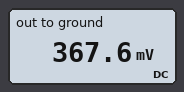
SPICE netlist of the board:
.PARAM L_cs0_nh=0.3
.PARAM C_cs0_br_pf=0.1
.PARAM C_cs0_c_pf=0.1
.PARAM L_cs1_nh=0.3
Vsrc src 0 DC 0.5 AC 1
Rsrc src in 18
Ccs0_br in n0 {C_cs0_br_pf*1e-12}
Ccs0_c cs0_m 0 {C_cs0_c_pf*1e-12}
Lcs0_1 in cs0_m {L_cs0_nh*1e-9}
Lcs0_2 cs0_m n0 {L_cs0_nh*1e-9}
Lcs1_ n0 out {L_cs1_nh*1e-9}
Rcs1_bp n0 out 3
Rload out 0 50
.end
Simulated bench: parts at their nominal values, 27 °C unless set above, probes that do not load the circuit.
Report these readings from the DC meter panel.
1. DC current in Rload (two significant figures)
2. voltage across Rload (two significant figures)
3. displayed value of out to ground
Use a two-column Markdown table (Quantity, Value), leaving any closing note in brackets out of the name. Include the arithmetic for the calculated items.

| Quantity | Value |
|---|---|
| DC current in Rload | (367.6 mV) / 50 Ω = 7.4 mA |
| voltage across Rload | 367.6 mV = 370 mV |
| displayed value of out to ground | 367.6 mV |
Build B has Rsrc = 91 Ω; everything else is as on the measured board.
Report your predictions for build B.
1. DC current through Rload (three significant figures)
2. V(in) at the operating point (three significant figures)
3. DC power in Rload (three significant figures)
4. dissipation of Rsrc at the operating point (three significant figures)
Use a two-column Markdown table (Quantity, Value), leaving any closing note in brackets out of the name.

| Quantity | Value |
|---|---|
| DC current through Rload | 3.55 mA |
| V(in) at the operating point | 177 mV |
| DC power in Rload | 629 µW |
| dissipation of Rsrc at the operating point | 1.14 mW |
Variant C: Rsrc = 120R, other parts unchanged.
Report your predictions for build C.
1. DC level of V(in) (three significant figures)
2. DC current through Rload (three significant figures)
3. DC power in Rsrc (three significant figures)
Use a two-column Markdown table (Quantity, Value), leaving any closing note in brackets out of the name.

| Quantity | Value |
|---|---|
| DC level of V(in) | 147 mV |
| DC current through Rload | 2.94 mA |
| DC power in Rsrc | 1.04 mW |
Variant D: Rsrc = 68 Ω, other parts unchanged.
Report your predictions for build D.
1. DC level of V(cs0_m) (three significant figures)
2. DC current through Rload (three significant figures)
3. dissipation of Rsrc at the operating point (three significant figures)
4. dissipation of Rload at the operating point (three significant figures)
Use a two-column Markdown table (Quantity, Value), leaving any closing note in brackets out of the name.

| Quantity | Value |
|---|---|
| DC level of V(cs0_m) | 212 mV |
| DC current through Rload | 4.24 mA |
| dissipation of Rsrc at the operating point | 1.22 mW |
| dissipation of Rload at the operating point | 898 µW |
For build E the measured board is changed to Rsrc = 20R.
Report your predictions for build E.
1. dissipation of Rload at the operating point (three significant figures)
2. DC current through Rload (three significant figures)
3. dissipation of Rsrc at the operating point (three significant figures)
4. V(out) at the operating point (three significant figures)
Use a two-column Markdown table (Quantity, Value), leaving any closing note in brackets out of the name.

| Quantity | Value |
|---|---|
| dissipation of Rload at the operating point | 2.55 mW |
| DC current through Rload | 7.14 mA |
| dissipation of Rsrc at the operating point | 1.02 mW |
| V(out) at the operating point | 357 mV |
